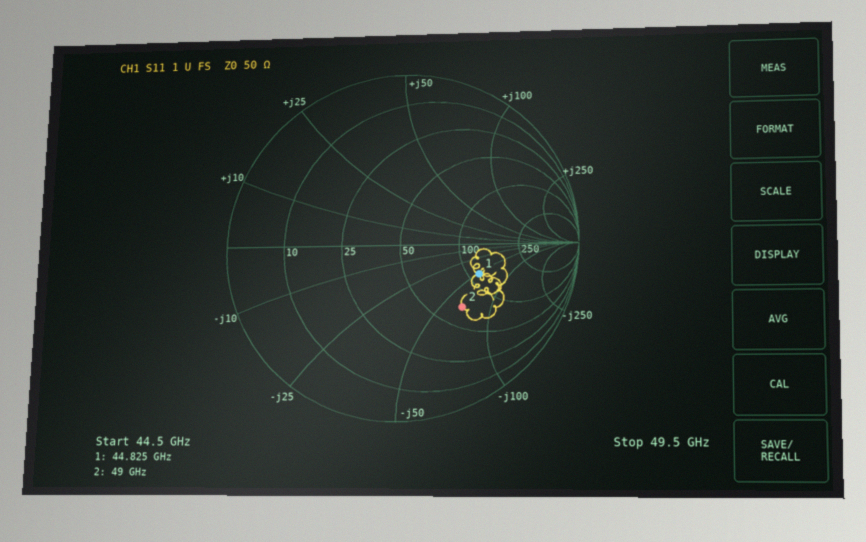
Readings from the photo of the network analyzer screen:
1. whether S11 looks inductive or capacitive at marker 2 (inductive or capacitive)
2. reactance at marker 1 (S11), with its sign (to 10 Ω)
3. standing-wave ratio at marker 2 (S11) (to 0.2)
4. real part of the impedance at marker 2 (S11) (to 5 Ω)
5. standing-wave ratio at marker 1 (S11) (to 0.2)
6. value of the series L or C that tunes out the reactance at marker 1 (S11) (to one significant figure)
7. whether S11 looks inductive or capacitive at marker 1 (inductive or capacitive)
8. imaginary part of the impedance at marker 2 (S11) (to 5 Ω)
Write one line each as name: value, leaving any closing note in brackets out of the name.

whether S11 looks inductive or capacitive at marker 2: capacitive
reactance at marker 1 (S11), with its sign: -50 Ω
standing-wave ratio at marker 2 (S11): 3.0
real part of the impedance at marker 2 (S11): 70 Ω
standing-wave ratio at marker 1 (S11): 2.8
value of the series L or C that tunes out the reactance at marker 1 (S11): 200 pH
whether S11 looks inductive or capacitive at marker 1: capacitive
imaginary part of the impedance at marker 2 (S11): -65 Ω
